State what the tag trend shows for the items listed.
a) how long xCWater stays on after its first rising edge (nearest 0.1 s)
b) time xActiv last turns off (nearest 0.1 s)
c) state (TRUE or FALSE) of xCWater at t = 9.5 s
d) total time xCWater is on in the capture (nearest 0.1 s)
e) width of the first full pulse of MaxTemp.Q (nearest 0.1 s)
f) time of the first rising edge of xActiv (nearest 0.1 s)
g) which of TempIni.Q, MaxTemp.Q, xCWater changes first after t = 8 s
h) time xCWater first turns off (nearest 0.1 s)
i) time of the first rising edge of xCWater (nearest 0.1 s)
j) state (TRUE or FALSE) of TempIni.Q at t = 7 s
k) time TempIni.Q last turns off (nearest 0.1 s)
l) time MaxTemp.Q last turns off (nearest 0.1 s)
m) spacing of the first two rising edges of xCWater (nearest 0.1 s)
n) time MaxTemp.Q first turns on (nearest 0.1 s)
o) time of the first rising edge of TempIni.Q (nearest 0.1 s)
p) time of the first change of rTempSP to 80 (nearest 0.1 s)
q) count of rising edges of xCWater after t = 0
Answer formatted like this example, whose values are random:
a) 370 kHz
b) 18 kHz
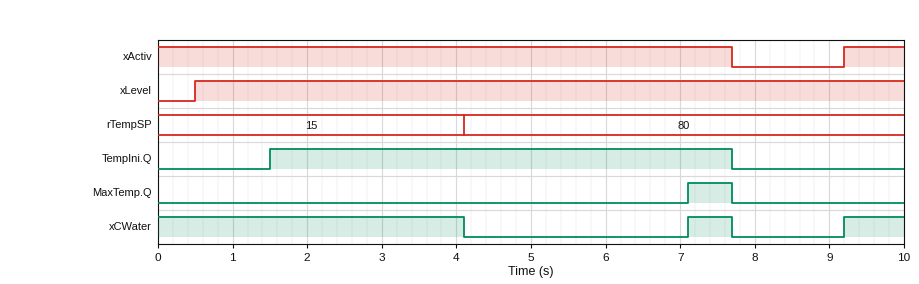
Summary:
a) 0.6 s
b) 7.7 s
c) TRUE
d) 5.5 s
e) 0.6 s
f) 9.2 s
g) xCWater
h) 4.1 s
i) 7.1 s
j) TRUE
k) 7.7 s
l) 7.7 s
m) 2.1 s
n) 7.1 s
o) 1.5 s
p) 4.1 s
q) 2
